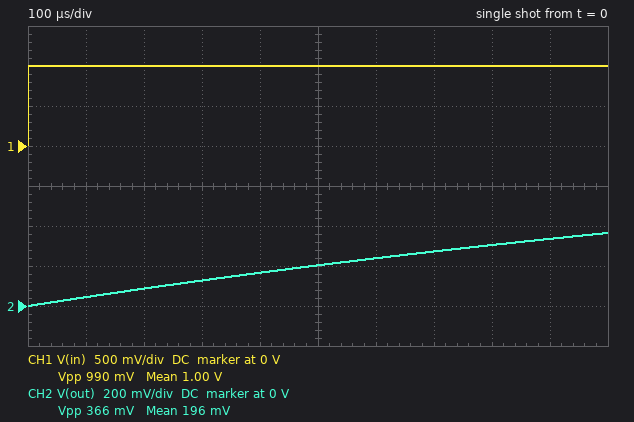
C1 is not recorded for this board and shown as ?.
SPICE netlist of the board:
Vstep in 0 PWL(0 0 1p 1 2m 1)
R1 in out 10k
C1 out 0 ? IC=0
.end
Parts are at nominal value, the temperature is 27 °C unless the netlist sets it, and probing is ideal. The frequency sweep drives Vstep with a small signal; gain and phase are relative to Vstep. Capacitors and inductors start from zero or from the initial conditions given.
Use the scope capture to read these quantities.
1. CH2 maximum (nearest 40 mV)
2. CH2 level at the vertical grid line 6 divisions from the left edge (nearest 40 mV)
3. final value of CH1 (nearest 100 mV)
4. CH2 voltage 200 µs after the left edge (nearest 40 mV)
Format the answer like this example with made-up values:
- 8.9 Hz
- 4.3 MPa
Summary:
- 360 mV
- 240 mV
- 1.0 V
- 80 mV
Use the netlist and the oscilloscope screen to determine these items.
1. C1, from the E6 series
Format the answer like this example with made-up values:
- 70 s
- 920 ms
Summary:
- 220 nF
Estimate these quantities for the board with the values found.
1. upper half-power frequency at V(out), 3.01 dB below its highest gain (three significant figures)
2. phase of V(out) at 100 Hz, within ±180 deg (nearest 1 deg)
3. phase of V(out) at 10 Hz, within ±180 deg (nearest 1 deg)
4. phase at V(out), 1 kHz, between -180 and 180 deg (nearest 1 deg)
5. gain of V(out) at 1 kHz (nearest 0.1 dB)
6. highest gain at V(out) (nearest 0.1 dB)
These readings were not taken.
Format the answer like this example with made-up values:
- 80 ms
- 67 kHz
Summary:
- 72.3 Hz
- -54 deg
- -8 deg
- -86 deg
- -22.8 dB
- 0 dB
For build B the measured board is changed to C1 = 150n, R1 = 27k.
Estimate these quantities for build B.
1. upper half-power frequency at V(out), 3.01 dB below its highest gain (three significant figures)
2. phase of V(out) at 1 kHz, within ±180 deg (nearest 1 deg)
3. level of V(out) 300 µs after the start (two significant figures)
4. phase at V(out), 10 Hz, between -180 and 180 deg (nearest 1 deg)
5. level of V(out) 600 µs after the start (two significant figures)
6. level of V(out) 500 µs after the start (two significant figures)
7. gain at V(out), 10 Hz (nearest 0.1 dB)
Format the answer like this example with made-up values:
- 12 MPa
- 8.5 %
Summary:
- 39.3 Hz
- -88 deg
- 71 mV
- -14 deg
- 140 mV
- 120 mV
- -0.3 dB
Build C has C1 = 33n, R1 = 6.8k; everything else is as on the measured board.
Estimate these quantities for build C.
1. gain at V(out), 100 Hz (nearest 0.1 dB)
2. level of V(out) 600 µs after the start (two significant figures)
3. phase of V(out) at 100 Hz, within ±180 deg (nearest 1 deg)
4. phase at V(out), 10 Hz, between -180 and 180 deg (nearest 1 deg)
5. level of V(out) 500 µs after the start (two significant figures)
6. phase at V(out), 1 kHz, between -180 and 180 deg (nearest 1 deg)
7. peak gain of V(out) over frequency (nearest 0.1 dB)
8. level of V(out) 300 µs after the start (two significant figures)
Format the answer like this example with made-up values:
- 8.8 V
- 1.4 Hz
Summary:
- -0.1 dB
- 930 mV
- -8 deg
- -1 deg
- 890 mV
- -55 deg
- 0 dB
- 740 mV
